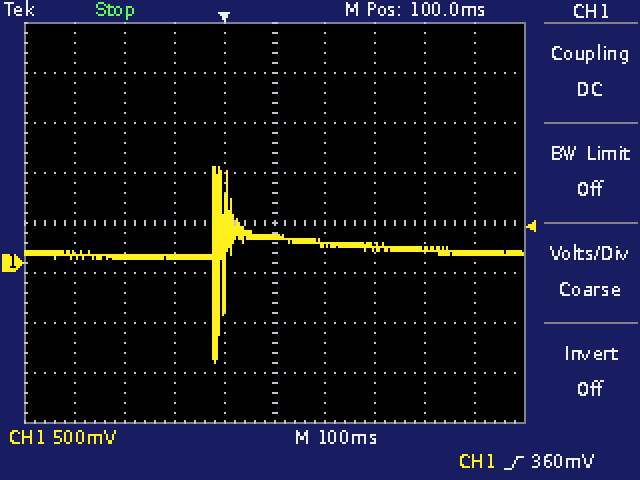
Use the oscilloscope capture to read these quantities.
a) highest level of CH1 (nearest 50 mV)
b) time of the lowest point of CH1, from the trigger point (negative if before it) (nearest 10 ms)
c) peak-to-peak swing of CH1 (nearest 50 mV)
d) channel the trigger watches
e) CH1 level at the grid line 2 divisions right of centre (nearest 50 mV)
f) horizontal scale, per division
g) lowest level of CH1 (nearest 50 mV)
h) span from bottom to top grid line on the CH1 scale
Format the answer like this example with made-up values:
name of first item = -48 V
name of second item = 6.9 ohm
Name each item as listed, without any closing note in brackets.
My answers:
highest level of CH1 = 950 mV
time of the lowest point of CH1, from the trigger point (negative if before it) = -20 ms
peak-to-peak swing of CH1 = 1.95 V
channel the trigger watches = CH1
CH1 level at the grid line 2 divisions right of centre = 150 mV
horizontal scale, per division = 100 ms
lowest level of CH1 = -1.00 V
span from bottom to top grid line on the CH1 scale = 4 V
